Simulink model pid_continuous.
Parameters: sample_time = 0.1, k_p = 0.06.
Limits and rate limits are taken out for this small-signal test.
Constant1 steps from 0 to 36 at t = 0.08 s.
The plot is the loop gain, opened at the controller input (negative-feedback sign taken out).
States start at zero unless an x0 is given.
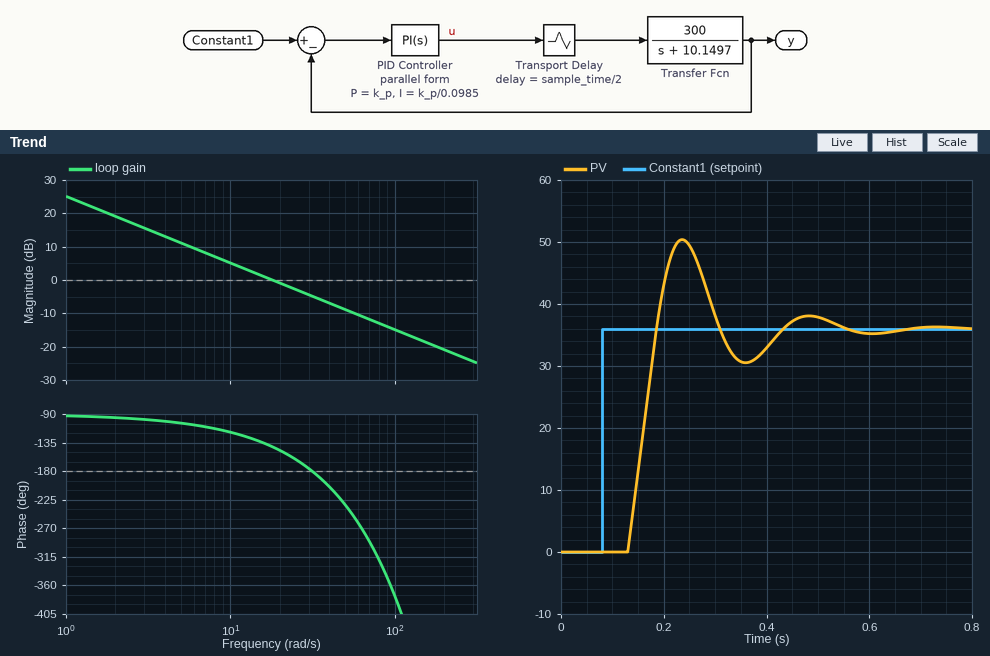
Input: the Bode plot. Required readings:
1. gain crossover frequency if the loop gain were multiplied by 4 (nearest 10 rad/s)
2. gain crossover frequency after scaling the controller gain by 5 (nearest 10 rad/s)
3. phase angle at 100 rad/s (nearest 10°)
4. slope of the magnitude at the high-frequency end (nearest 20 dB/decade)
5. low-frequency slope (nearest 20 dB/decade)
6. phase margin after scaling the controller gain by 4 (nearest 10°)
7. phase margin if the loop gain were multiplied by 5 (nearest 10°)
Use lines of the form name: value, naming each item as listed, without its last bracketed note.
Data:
gain crossover frequency if the loop gain were multiplied by 4: 70 rad/s
gain crossover frequency after scaling the controller gain by 5: 90 rad/s
phase angle at 100 rad/s: -380°
slope of the magnitude at the high-frequency end: -20 dB/decade
low-frequency slope: -20 dB/decade
phase margin after scaling the controller gain by 4: -120°
phase margin if the loop gain were multiplied by 5: -170°
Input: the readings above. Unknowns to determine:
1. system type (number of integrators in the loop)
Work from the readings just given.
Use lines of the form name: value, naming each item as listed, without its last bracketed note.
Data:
system type: 1
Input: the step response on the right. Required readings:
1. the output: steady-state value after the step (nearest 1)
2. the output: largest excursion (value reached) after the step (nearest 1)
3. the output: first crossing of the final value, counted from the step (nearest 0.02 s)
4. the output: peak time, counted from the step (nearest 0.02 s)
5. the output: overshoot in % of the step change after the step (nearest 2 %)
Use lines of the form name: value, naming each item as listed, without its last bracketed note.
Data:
the output: steady-state value after the step: 36
the output: largest excursion (value reached) after the step: 50
the output: first crossing of the final value, counted from the step: 0.10 s
the output: peak time, counted from the step: 0.16 s
the output: overshoot in % of the step change after the step: 40 %
